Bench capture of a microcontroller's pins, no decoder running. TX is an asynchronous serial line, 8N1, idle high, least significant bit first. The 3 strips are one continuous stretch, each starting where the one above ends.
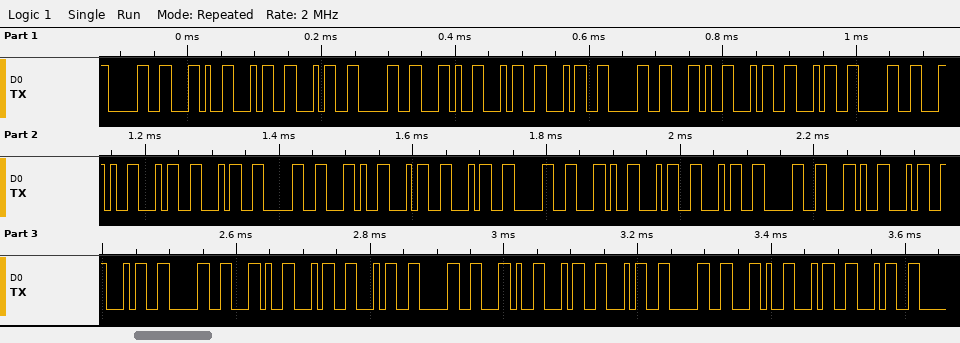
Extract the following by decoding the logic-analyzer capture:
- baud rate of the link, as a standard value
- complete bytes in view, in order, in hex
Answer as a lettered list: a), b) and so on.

a) 115200 baud
b) 30 2C 34 34 30 2C 34 34 30 2C 34 34 30 2C 34 34 30 2C 34 34 30 2C 34 34 30 2C 34 34 30 2C 34 34 30 2C 34 34 30 2C 34 34
